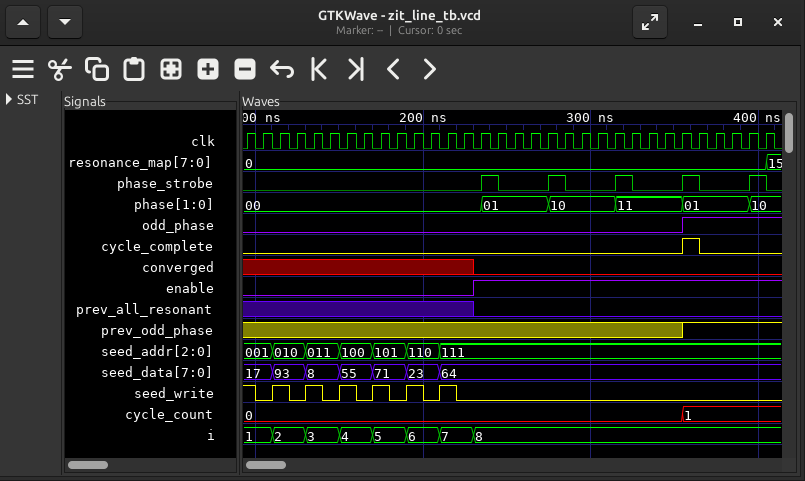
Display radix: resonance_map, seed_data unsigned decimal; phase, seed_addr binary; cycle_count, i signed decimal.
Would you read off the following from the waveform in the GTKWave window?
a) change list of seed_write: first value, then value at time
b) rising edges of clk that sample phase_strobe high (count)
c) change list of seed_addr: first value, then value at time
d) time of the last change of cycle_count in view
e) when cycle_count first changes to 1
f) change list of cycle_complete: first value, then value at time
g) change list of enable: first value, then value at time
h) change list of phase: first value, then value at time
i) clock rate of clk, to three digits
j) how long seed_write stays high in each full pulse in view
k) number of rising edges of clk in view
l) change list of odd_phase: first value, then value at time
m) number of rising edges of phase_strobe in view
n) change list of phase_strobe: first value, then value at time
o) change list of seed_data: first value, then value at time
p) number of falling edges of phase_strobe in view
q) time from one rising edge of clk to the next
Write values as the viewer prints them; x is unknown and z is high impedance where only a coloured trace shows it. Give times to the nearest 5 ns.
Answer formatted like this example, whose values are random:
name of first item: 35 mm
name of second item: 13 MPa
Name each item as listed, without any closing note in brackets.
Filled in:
change list of seed_write: first value, then value at time: 1, 0 at 100 ns, 1 at 110 ns, 0 at 120 ns, 1 at 130 ns, 0 at 140 ns, 1 at 150 ns, 0 at 160 ns, 1 at 170 ns, 0 at 180 ns, 1 at 190 ns, 0 at 200 ns, 1 at 210 ns, 0 at 220 ns
rising edges of clk that sample phase_strobe high: 5
change list of seed_addr: first value, then value at time: 001, 010 at 110 ns, 011 at 130 ns, 100 at 150 ns, 101 at 170 ns, 110 at 190 ns, 111 at 210 ns
time of the last change of cycle_count in view: 355 ns
when cycle_count first changes to 1: 355 ns
change list of cycle_complete: first value, then value at time: 0, 1 at 355 ns, 0 at 365 ns
change list of enable: first value, then value at time: 0, 1 at 230 ns
change list of phase: first value, then value at time: 00, 01 at 235 ns, 10 at 275 ns, 11 at 315 ns, 01 at 355 ns, 10 at 395 ns
clock rate of clk, to three digits: 100 MHz
how long seed_write stays high in each full pulse in view: 10 ns, 10 ns, 10 ns, 10 ns, 10 ns, 10 ns
number of rising edges of clk in view: 32
change list of odd_phase: first value, then value at time: 0, 1 at 355 ns
number of rising edges of phase_strobe in view: 5
change list of phase_strobe: first value, then value at time: 0, 1 at 235 ns, 0 at 245 ns, 1 at 275 ns, 0 at 285 ns, 1 at 315 ns, 0 at 325 ns, 1 at 355 ns, 0 at 365 ns, 1 at 395 ns, 0 at 405 ns
change list of seed_data: first value, then value at time: 17, 93 at 110 ns, 8 at 130 ns, 55 at 150 ns, 71 at 170 ns, 23 at 190 ns, 64 at 210 ns
number of falling edges of phase_strobe in view: 5
time from one rising edge of clk to the next: 10 ns
